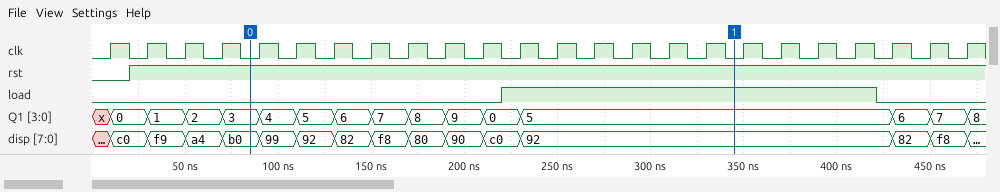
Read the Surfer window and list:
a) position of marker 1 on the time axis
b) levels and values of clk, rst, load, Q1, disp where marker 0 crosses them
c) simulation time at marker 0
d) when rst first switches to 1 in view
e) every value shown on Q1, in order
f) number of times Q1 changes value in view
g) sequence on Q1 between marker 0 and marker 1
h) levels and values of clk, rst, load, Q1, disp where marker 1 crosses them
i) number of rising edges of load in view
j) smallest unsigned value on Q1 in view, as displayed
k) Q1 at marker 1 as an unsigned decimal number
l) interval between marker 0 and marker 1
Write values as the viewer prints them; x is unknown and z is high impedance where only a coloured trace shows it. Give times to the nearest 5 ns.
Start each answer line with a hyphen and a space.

- 345 ns
- clk=0, rst=1, load=0, Q1=3, disp=b0
- 85 ns
- 20 ns
- x, 0, 1, 2, 3, 4, 5, 6, 7, 8, 9, 0, 5, 6, 7, 8
- 15
- 3, 4, 5, 6, 7, 8, 9, 0, 5
- clk=0, rst=1, load=1, Q1=5, disp=92
- 1
- 0
- 5
- 260 ns
